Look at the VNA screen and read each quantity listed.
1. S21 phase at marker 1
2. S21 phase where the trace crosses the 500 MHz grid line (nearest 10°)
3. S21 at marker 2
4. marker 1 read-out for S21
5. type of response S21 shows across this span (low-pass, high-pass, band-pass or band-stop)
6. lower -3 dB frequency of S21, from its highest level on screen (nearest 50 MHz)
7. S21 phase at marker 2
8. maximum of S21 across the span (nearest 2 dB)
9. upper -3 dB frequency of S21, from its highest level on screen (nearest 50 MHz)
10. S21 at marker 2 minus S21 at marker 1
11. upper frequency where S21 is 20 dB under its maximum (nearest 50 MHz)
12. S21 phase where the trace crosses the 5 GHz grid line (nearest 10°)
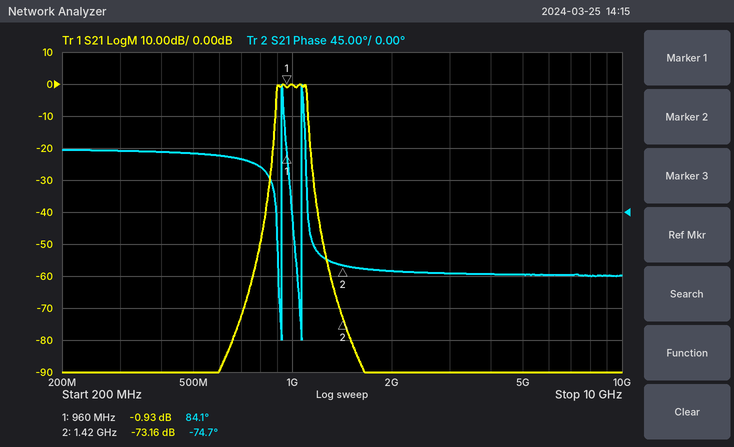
84.1°
80°
-73.16 dB
-0.93 dB
band-pass
900 MHz
-74.7°
0 dB
1.10 GHz
-72.23 dB
1.15 GHz
-90°
